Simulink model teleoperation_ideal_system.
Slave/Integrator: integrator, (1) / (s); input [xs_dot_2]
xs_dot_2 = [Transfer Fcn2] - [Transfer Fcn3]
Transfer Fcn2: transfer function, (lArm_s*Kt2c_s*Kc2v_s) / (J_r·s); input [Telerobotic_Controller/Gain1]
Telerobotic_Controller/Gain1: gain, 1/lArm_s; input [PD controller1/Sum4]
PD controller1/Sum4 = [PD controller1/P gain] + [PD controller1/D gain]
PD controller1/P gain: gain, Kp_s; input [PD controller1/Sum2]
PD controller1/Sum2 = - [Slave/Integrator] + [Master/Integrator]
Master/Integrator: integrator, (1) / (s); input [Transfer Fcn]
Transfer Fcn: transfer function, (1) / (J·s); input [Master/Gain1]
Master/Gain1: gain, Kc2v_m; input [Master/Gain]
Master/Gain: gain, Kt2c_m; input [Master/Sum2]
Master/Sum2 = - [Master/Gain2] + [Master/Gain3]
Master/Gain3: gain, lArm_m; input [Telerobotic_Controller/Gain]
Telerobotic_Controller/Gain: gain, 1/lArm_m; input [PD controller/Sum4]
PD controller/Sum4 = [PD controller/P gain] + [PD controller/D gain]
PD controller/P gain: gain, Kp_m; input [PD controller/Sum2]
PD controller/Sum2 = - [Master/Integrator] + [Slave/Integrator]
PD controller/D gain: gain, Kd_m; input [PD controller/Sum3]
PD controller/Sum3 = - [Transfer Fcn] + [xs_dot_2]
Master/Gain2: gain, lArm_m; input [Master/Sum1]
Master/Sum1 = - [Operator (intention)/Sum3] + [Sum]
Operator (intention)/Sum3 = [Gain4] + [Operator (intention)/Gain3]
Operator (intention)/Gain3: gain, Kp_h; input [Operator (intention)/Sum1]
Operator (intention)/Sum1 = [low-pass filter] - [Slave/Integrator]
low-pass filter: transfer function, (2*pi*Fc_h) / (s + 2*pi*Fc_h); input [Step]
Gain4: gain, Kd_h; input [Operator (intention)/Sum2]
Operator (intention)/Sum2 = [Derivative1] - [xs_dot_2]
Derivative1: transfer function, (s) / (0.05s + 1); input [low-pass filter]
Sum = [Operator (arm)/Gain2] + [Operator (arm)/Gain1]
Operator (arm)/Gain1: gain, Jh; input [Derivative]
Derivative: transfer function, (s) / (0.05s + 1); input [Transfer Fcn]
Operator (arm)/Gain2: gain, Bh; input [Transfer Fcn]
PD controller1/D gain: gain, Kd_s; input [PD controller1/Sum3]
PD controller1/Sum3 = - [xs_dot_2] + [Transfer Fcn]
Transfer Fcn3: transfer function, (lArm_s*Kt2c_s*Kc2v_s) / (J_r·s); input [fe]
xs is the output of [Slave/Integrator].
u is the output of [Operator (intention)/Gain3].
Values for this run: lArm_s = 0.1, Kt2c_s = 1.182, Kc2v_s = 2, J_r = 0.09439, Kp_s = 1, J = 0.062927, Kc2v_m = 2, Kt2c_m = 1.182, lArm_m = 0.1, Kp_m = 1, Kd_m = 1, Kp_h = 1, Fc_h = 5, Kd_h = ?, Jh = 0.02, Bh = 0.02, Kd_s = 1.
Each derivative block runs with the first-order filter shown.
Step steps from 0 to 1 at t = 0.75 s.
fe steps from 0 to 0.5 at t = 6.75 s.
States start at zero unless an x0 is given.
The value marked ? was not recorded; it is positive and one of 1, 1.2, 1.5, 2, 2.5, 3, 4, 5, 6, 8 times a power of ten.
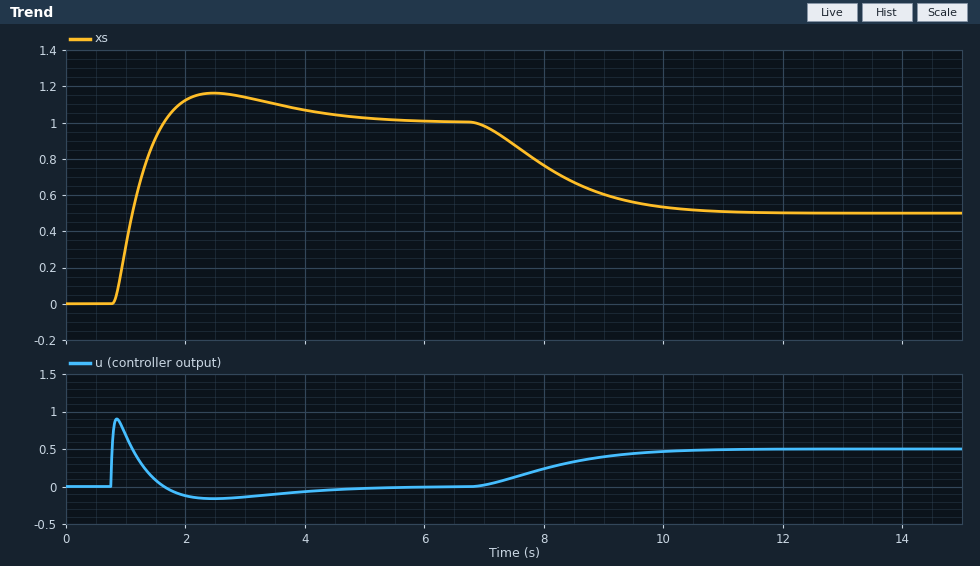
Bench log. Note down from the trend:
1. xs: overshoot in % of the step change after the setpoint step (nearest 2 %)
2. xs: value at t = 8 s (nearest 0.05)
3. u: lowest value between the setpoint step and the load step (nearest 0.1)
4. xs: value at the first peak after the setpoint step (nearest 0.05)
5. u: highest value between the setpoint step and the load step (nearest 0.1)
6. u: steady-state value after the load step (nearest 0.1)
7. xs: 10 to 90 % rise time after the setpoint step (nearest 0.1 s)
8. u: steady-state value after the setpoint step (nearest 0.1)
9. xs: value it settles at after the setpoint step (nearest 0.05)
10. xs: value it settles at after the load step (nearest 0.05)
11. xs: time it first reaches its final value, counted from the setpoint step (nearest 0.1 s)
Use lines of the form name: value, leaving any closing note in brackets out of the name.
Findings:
xs: overshoot in % of the step change after the setpoint step: 16 %
xs: value at t = 8 s: 0.75
u: lowest value between the setpoint step and the load step: -0.2
xs: value at the first peak after the setpoint step: 1.15
u: highest value between the setpoint step and the load step: 0.9
u: steady-state value after the load step: 0.5
xs: 10 to 90 % rise time after the setpoint step: 0.6 s
u: steady-state value after the setpoint step: 0.0
xs: value it settles at after the setpoint step: 1.00
xs: value it settles at after the load step: 0.50
xs: time it first reaches its final value, counted from the setpoint step: 0.9 s
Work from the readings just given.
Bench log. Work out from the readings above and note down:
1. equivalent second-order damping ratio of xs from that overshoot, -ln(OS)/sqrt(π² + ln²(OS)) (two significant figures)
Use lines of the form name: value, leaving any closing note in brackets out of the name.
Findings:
equivalent second-order damping ratio of xs from that overshoot, -ln(OS)/sqrt(π² + ln²(OS)): 0.50
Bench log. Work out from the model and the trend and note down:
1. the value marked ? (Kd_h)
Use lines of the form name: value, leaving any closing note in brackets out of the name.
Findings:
the value marked ?: 1.5
